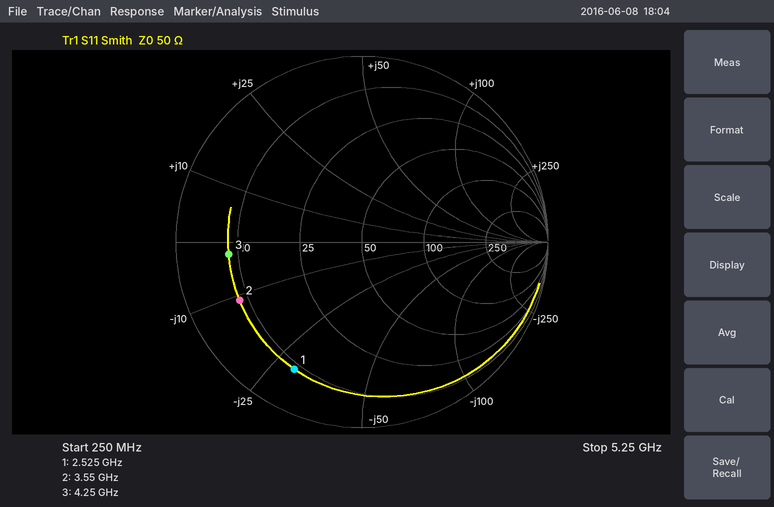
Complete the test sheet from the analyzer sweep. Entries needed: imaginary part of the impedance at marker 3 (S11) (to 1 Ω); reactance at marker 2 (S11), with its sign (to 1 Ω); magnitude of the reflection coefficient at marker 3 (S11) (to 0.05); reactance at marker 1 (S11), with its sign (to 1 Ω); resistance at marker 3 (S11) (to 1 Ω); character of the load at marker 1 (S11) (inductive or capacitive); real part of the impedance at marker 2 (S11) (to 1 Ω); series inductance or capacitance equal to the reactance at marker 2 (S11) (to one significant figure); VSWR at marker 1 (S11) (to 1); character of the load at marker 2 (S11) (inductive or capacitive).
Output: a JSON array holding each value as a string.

["-2 Ω", "-11 Ω", "0.70", "-29 Ω", "8 Ω", "capacitive", "8 Ω", "4 pF", "8", "capacitive"]
